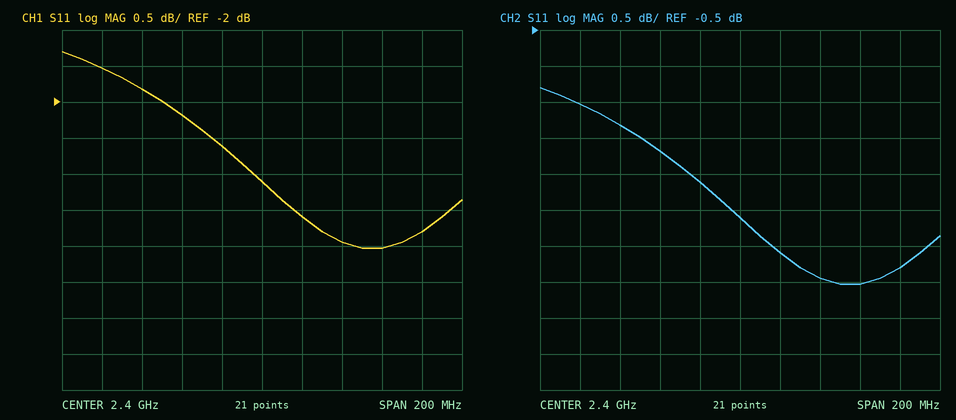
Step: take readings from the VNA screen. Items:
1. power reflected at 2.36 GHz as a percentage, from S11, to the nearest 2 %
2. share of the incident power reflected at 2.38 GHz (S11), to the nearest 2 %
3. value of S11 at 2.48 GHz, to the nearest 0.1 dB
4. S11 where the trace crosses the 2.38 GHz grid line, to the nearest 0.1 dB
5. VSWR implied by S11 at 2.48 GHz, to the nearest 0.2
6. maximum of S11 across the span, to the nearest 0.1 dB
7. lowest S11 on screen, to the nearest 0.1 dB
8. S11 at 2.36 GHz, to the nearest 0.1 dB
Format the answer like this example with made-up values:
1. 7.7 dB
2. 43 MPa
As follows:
1. 60 %
2. 54 %
3. -3.8 dB
4. -2.6 dB
5. 4.6
6. -1.3 dB
7. -4.0 dB
8. -2.2 dB
